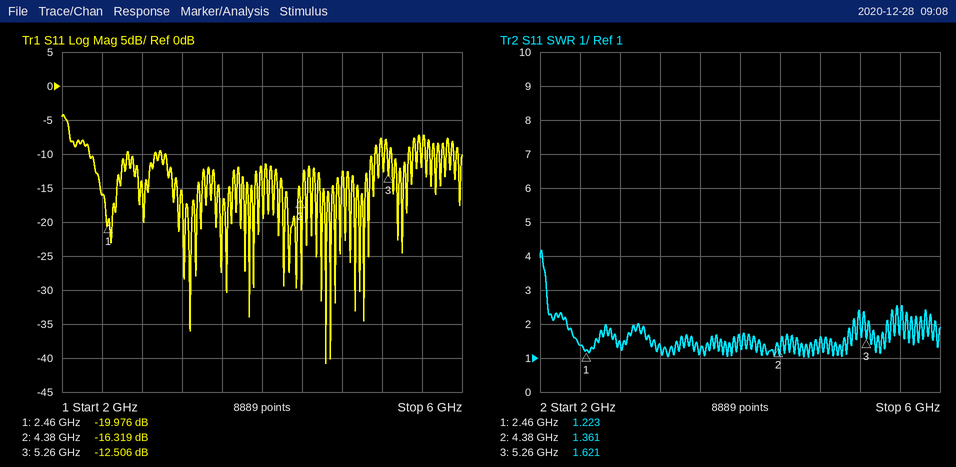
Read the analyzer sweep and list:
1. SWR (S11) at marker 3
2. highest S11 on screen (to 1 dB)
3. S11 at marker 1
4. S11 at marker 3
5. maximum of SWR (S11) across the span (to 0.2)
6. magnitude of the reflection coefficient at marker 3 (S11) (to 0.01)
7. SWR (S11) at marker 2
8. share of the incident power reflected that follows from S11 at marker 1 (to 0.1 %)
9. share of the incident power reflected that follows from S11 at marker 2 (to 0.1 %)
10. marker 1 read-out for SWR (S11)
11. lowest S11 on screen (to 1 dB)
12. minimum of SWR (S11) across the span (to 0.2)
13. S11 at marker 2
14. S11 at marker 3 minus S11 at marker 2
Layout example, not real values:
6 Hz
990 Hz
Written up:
1.621
-4 dB
-19.976 dB
-12.506 dB
4.2
0.24
1.361
1.0 %
2.3 %
1.223
-41 dB
1.0
-16.319 dB
3.813 dB
